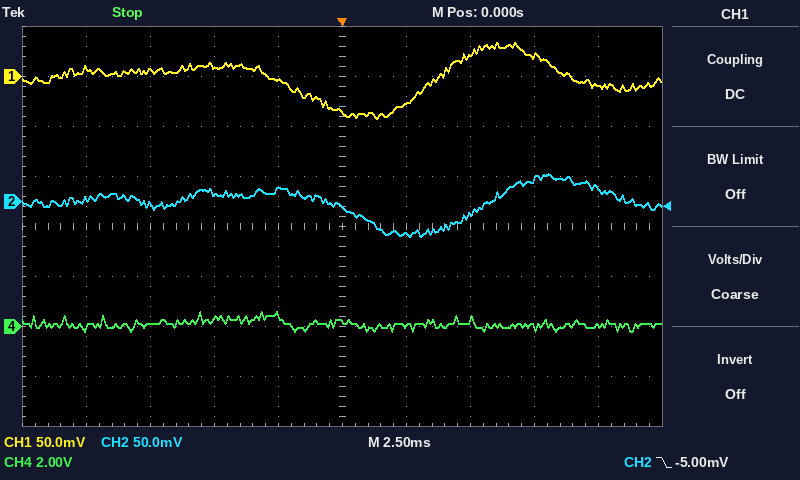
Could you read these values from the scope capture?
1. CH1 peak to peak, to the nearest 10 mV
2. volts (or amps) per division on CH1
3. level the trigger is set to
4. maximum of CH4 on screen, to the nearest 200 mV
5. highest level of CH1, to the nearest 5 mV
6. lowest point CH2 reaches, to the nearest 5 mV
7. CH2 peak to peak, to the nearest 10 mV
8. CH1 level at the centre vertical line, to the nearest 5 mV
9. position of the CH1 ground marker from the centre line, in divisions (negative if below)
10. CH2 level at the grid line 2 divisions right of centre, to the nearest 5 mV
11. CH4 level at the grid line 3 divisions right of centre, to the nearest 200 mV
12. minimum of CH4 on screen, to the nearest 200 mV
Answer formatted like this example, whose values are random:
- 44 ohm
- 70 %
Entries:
- 80 mV
- 50 mV
- -5.00 mV
- 600 mV
- 35 mV
- -35 mV
- 60 mV
- -35 mV
- +3.0 div
- -15 mV
- 0.0 V
- -200 mV
